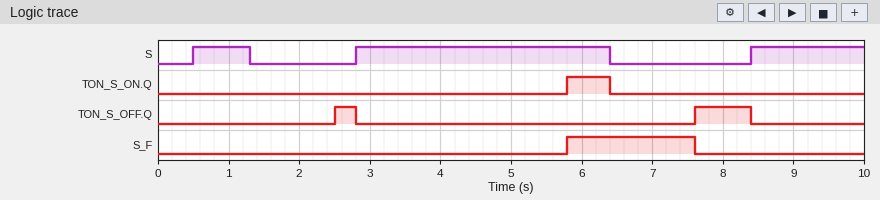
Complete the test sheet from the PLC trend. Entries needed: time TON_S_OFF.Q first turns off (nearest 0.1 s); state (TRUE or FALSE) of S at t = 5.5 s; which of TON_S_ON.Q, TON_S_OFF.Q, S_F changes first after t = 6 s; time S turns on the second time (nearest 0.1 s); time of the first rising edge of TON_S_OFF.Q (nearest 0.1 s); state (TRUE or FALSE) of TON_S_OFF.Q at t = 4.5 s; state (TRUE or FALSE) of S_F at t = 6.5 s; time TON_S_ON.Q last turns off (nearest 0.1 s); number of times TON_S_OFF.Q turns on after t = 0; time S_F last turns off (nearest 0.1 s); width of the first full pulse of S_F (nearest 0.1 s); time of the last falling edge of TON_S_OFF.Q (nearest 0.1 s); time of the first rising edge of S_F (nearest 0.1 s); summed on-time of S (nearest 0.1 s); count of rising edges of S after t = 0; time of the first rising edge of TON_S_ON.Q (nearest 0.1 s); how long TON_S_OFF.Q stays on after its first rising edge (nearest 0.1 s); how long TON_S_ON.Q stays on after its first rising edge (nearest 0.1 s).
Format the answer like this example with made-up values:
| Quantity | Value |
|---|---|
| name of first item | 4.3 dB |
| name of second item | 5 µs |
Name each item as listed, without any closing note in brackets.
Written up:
| Quantity | Value |
|---|---|
| time TON_S_OFF.Q first turns off | 2.8 s |
| state (TRUE or FALSE) of S at t = 5.5 s | TRUE |
| which of TON_S_ON.Q, TON_S_OFF.Q, S_F changes first after t = 6 s | TON_S_ON.Q |
| time S turns on the second time | 2.8 s |
| time of the first rising edge of TON_S_OFF.Q | 2.5 s |
| state (TRUE or FALSE) of TON_S_OFF.Q at t = 4.5 s | FALSE |
| state (TRUE or FALSE) of S_F at t = 6.5 s | TRUE |
| time TON_S_ON.Q last turns off | 6.4 s |
| number of times TON_S_OFF.Q turns on after t = 0 | 2 |
| time S_F last turns off | 7.6 s |
| width of the first full pulse of S_F | 1.8 s |
| time of the last falling edge of TON_S_OFF.Q | 8.4 s |
| time of the first rising edge of S_F | 5.8 s |
| summed on-time of S | 6.0 s |
| count of rising edges of S after t = 0 | 3 |
| time of the first rising edge of TON_S_ON.Q | 5.8 s |
| how long TON_S_OFF.Q stays on after its first rising edge | 0.3 s |
| how long TON_S_ON.Q stays on after its first rising edge | 0.6 s |
